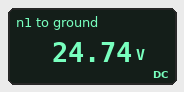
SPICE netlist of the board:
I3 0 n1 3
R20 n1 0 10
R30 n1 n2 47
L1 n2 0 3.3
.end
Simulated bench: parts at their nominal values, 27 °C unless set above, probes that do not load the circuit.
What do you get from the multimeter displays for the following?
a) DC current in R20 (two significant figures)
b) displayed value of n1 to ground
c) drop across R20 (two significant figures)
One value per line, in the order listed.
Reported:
2.5 A
24.74 V
25 V
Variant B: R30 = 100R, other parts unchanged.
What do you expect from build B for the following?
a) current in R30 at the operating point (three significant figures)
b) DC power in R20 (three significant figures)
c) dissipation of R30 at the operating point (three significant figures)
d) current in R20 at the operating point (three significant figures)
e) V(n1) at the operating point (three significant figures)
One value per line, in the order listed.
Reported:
273 mA
74.4 W
7.44 W
2.73 A
27.3 V
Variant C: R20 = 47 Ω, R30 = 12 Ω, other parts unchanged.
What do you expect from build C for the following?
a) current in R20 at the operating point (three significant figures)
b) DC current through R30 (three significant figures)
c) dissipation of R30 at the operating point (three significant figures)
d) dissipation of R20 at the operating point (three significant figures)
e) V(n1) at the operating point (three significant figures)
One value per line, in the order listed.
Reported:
610 mA
2.39 A
68.5 W
17.5 W
28.7 V
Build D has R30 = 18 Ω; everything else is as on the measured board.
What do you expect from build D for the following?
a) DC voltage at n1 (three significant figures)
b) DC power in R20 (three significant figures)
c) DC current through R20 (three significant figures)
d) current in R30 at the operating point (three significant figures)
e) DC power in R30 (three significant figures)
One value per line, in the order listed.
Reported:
19.3 V
37.2 W
1.93 A
1.07 A
20.7 W
